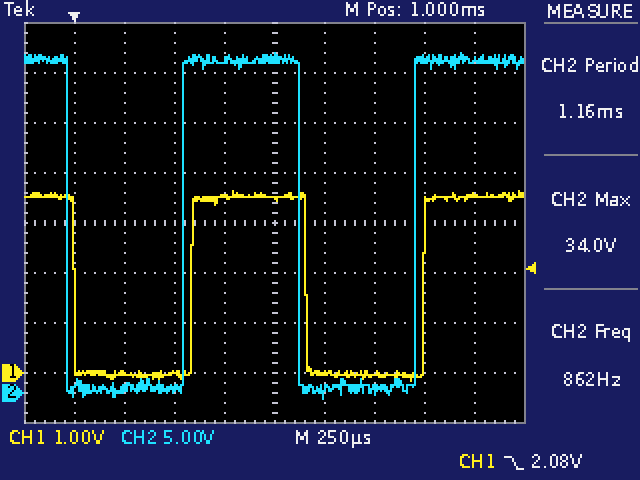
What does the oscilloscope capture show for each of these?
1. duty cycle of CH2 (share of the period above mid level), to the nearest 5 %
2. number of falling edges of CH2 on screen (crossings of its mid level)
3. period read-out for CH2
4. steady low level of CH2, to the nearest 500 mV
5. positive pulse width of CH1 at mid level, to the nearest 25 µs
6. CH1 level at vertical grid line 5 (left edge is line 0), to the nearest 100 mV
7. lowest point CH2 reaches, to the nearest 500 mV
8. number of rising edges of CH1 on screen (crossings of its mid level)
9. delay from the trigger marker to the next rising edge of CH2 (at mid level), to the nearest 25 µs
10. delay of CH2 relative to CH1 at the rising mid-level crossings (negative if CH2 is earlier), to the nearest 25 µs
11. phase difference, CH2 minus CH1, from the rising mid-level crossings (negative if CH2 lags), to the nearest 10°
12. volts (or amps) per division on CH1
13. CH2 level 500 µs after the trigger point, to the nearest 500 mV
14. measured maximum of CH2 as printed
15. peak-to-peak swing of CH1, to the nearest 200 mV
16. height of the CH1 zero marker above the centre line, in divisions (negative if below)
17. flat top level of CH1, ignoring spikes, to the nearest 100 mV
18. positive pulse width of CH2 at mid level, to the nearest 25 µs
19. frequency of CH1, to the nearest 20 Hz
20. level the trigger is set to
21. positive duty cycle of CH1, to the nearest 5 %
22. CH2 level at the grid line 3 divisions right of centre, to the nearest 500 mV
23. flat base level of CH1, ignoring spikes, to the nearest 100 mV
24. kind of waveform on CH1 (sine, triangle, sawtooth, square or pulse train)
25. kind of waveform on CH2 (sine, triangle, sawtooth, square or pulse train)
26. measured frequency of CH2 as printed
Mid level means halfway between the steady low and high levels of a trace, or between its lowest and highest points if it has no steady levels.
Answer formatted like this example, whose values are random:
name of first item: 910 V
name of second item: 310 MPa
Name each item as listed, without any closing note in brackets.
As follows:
duty cycle of CH2 (share of the period above mid level), to the nearest 5 %: 50 %
number of falling edges of CH2 on screen: 2
period read-out for CH2: 1.16 ms
steady low level of CH2, to the nearest 500 mV: 500 mV
positive pulse width of CH1 at mid level, to the nearest 25 µs: 575 µs
CH1 level at vertical grid line 5 (left edge is line 0), to the nearest 100 mV: 3.5 V
lowest point CH2 reaches, to the nearest 500 mV: -500 mV
number of rising edges of CH1 on screen: 2
delay from the trigger marker to the next rising edge of CH2 (at mid level), to the nearest 25 µs: 550 µs
delay of CH2 relative to CH1 at the rising mid-level crossings (negative if CH2 is earlier), to the nearest 25 µs: -50 µs
phase difference, CH2 minus CH1, from the rising mid-level crossings (negative if CH2 lags), to the nearest 10°: +10°
volts (or amps) per division on CH1: 1 V
CH2 level 500 µs after the trigger point, to the nearest 500 mV: 500 mV
measured maximum of CH2 as printed: 34.0 V
peak-to-peak swing of CH1, to the nearest 200 mV: 3.8 V
height of the CH1 zero marker above the centre line, in divisions: -3.0 div
flat top level of CH1, ignoring spikes, to the nearest 100 mV: 3.5 V
positive pulse width of CH2 at mid level, to the nearest 25 µs: 575 µs
frequency of CH1, to the nearest 20 Hz: 860 Hz
level the trigger is set to: 2.08 V
positive duty cycle of CH1, to the nearest 5 %: 50 %
CH2 level at the grid line 3 divisions right of centre, to the nearest 500 mV: 33.5 V
flat base level of CH1, ignoring spikes, to the nearest 100 mV: 0.0 V
kind of waveform on CH1: square
kind of waveform on CH2: square
measured frequency of CH2 as printed: 862 Hz
